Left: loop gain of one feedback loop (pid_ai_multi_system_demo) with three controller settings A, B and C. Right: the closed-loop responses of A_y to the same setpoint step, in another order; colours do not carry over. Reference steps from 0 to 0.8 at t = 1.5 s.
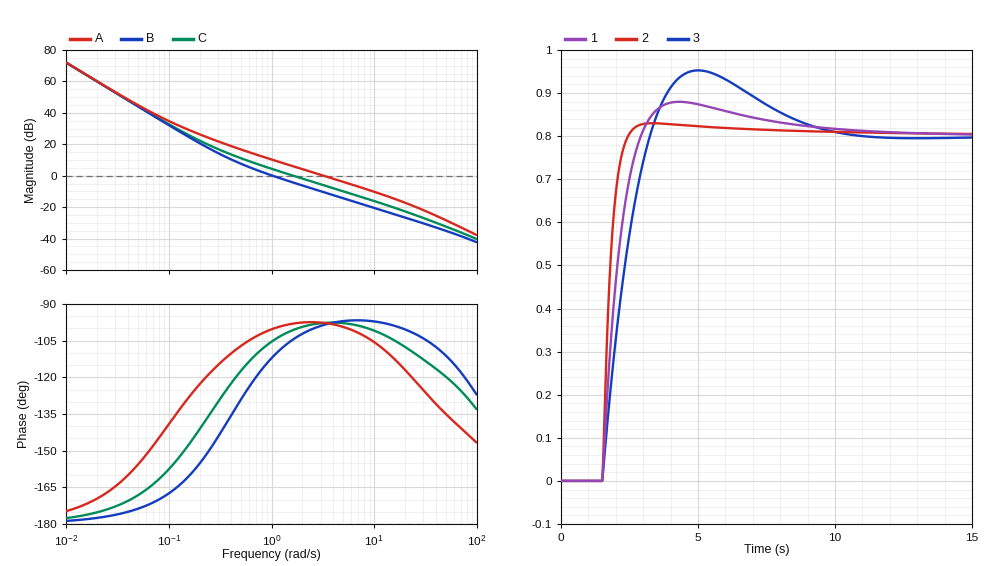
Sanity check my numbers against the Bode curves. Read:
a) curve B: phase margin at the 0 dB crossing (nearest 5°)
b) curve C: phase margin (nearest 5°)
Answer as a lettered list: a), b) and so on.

a) 70°
b) 80°
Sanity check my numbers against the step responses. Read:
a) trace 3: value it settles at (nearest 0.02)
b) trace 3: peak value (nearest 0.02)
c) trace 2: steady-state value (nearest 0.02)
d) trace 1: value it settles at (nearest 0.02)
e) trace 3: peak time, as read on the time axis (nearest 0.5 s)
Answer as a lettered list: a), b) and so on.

a) 0.80
b) 0.96
c) 0.80
d) 0.80
e) 5.0 s
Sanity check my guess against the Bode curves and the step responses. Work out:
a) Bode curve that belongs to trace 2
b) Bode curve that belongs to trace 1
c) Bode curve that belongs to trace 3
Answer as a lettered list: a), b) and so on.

a) A
b) C
c) B
